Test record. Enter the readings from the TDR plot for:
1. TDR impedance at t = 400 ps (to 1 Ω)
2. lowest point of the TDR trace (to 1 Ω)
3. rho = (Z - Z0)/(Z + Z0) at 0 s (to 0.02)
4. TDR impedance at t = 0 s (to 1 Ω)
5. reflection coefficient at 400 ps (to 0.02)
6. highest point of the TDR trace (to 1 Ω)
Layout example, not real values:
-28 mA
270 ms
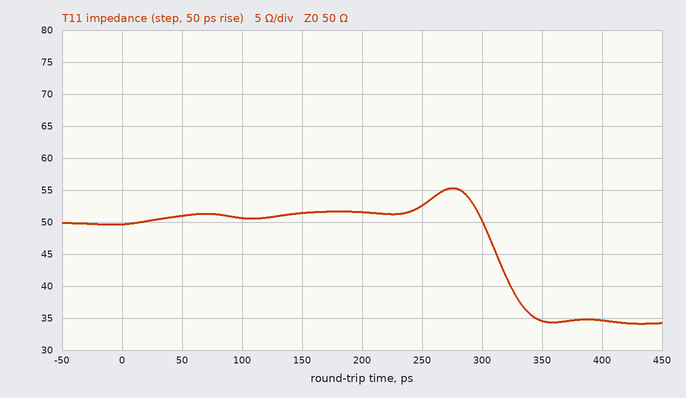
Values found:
35 Ω
34 Ω
0.00
50 Ω
-0.18
55 Ω
